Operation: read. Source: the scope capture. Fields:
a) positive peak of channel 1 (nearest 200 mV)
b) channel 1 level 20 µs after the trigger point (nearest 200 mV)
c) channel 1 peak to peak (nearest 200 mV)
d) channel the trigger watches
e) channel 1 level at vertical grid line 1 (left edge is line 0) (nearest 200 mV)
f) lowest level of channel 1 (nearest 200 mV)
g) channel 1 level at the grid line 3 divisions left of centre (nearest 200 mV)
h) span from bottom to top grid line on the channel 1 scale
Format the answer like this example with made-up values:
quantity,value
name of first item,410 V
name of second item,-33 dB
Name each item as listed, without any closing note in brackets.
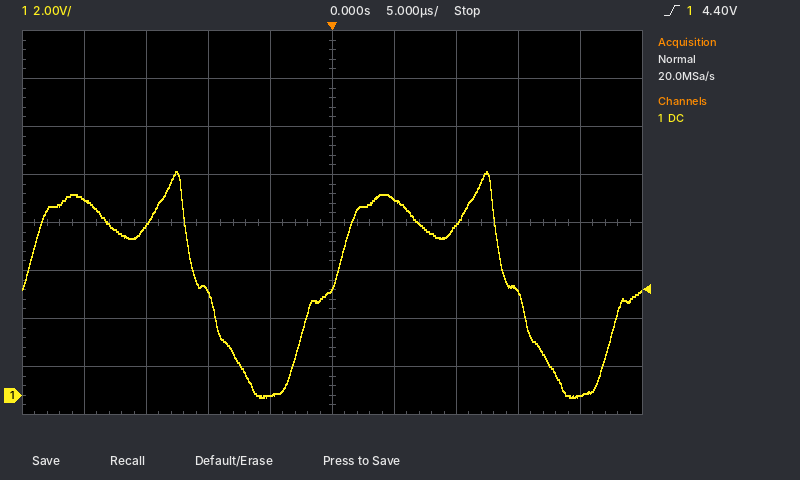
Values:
quantity,value
positive peak of channel 1,9.4 V
channel 1 level 20 µs after the trigger point,0.0 V
channel 1 peak to peak,9.4 V
channel the trigger watches,channel 1
channel 1 level at vertical grid line 1 (left edge is line 0),8.2 V
lowest level of channel 1,0.0 V
channel 1 level at the grid line 3 divisions left of centre,7.0 V
span from bottom to top grid line on the channel 1 scale,16 V
